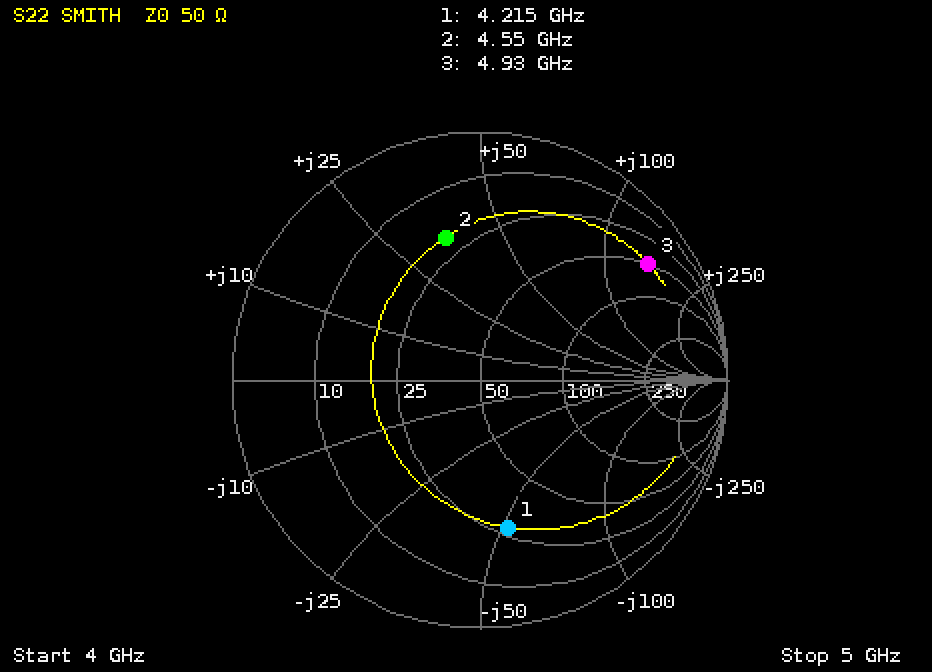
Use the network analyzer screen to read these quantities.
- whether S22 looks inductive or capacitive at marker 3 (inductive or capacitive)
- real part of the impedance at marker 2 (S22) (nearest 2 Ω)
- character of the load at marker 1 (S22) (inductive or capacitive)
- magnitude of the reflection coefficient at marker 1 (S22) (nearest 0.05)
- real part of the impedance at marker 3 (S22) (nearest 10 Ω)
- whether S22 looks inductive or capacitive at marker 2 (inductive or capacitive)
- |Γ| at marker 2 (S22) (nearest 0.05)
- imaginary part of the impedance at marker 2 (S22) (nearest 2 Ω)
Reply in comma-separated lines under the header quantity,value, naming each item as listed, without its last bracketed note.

quantity,value
whether S22 looks inductive or capacitive at marker 3,inductive
real part of the impedance at marker 2 (S22),20 Ω
character of the load at marker 1 (S22),capacitive
magnitude of the reflection coefficient at marker 1 (S22),0.60
real part of the impedance at marker 3 (S22),50 Ω
whether S22 looks inductive or capacitive at marker 2,inductive
|Γ| at marker 2 (S22),0.60
imaginary part of the impedance at marker 2 (S22),+36 Ω
